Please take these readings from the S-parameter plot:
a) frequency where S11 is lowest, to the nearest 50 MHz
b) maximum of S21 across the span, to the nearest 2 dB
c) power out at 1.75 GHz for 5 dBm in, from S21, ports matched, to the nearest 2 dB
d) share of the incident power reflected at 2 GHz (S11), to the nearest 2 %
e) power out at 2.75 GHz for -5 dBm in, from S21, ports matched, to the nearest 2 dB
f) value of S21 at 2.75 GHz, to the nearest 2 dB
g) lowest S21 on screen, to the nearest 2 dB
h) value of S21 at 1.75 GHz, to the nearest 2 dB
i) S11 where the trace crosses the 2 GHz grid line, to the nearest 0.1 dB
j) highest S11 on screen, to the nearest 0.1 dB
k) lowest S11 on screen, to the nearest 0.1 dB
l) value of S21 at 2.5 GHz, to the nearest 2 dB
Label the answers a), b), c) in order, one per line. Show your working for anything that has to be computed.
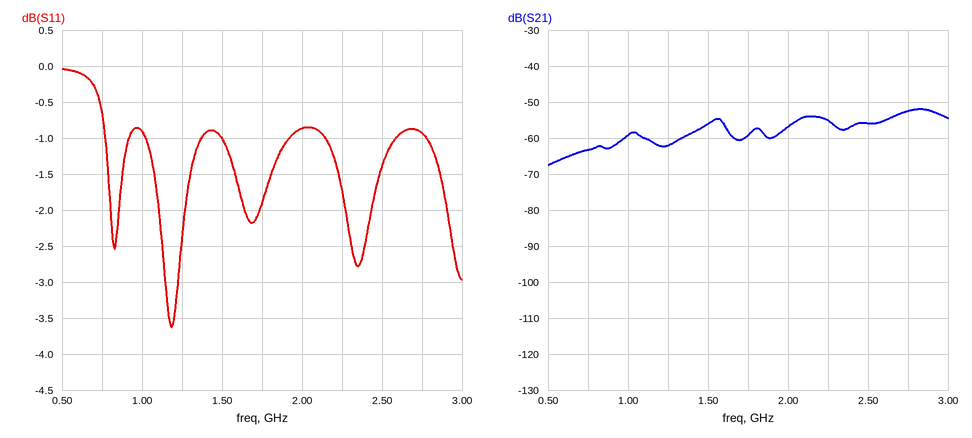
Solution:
a) 1.20 GHz
b) -52 dB
c) 5 dBm + (-60 dB) = -54 dBm
d) 10^(-0.9/10) ≈ 81.3 %, so 82 % to the nearest 2 %
e) -5 dBm + (-52 dB) = -58 dBm
f) -52 dB
g) -68 dB
h) -60 dB
i) -0.9 dB
j) 0.0 dB
k) -3.6 dB
l) -56 dB
